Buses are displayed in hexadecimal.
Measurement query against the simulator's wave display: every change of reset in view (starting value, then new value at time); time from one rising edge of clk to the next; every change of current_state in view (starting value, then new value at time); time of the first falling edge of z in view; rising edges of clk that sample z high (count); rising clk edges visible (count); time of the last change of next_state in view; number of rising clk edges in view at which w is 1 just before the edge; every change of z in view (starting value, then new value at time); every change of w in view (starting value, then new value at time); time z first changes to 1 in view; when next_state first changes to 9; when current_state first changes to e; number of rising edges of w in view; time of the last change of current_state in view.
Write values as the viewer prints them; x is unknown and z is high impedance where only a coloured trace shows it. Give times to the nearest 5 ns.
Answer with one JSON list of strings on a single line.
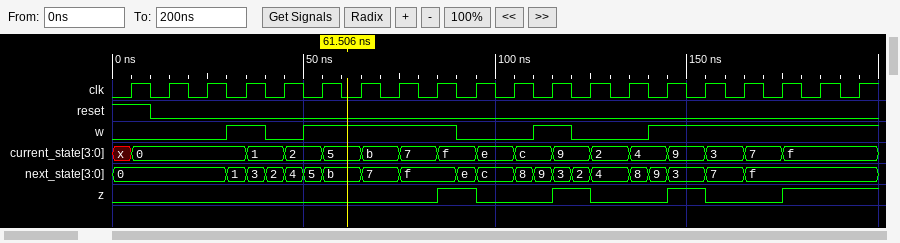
["1, 0 at 10 ns", "10 ns", "x, 0 at 5 ns, 1 at 35 ns, 2 at 45 ns, 5 at 55 ns, b at 65 ns, 7 at 75 ns, f at 85 ns, e at 95 ns, c at 105 ns, 9 at 115 ns, 2 at 125 ns, 4 at 135 ns, 9 at 145 ns, 3 at 155 ns, 7 at 165 ns, f at 175 ns", "95 ns", "5", "20", "165 ns", "12", "0, 1 at 85 ns, 0 at 95 ns, 1 at 115 ns, 0 at 125 ns, 1 at 145 ns, 0 at 155 ns, 1 at 175 ns", "0, 1 at 30 ns, 0 at 40 ns, 1 at 50 ns, 0 at 90 ns, 1 at 110 ns, 0 at 120 ns, 1 at 140 ns", "85 ns", "110 ns", "95 ns", "4", "175 ns"]
